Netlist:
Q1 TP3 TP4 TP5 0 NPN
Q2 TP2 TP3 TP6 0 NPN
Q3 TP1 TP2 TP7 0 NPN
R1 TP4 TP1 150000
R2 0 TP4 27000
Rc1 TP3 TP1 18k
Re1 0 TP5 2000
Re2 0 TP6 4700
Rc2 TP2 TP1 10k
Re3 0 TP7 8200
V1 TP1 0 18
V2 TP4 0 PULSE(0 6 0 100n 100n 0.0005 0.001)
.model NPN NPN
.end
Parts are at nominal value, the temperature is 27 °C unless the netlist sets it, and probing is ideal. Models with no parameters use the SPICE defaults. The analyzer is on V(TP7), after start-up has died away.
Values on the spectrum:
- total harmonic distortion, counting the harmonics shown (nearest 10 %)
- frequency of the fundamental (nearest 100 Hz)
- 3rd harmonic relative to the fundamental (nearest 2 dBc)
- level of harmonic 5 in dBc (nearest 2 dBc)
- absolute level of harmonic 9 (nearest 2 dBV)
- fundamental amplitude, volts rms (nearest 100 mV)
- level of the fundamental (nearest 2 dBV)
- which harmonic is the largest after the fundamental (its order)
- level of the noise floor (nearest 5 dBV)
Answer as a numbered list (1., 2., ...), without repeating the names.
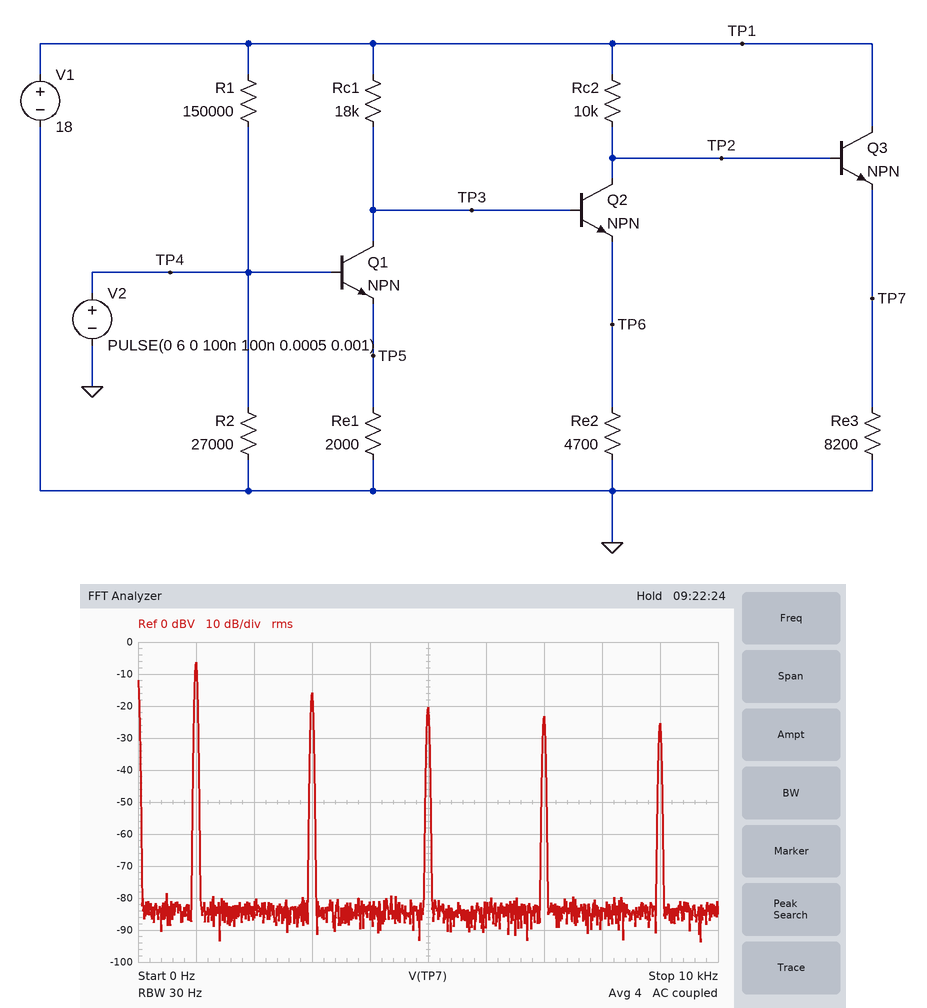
1. 40 %
2. 1.0 kHz
3. -10 dBc
4. -14 dBc
5. -26 dBV
6. 500 mV
7. -6 dBV
8. 3
9. -85 dBV
